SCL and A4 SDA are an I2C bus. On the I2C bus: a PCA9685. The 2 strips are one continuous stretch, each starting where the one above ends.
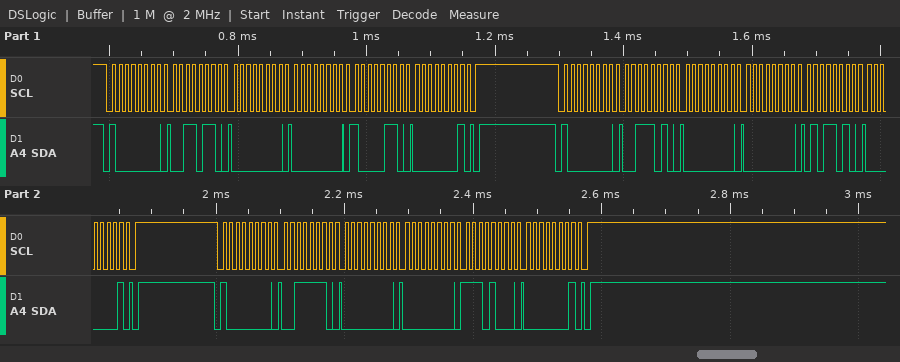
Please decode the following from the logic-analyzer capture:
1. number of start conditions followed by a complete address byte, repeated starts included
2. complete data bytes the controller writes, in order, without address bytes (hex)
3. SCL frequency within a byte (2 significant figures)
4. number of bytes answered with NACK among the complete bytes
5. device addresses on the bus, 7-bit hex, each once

3
36 00 00 86 01 3A 00 00 5A 01 3E 00 00 E8 01
100 kHz
0
0x40
